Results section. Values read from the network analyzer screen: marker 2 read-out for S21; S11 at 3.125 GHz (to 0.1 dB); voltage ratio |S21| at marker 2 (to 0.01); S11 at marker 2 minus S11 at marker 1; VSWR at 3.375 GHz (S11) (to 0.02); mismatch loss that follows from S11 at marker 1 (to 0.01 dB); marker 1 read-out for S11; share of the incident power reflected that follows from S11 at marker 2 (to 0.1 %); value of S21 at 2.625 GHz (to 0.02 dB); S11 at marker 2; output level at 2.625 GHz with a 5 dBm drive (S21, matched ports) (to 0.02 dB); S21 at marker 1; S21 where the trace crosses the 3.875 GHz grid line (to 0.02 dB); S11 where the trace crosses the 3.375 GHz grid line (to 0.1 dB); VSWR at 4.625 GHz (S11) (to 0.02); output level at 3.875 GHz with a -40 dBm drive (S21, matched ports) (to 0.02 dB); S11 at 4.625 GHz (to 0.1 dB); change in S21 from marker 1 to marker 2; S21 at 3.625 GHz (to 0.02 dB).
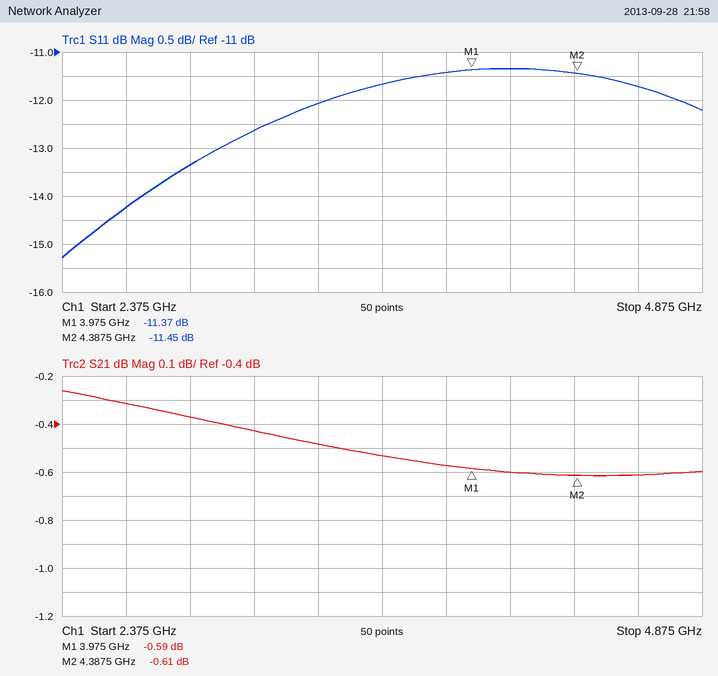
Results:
-0.61 dB
-12.6 dB
0.93
-0.08 dB
1.66
0.33 dB
-11.37 dB
7.2 %
-0.32 dB
-11.45 dB
4.68 dBm
-0.59 dB
-0.58 dB
-12.1 dB
1.70
-40.58 dBm
-11.7 dB
-0.02 dB
-0.54 dB
